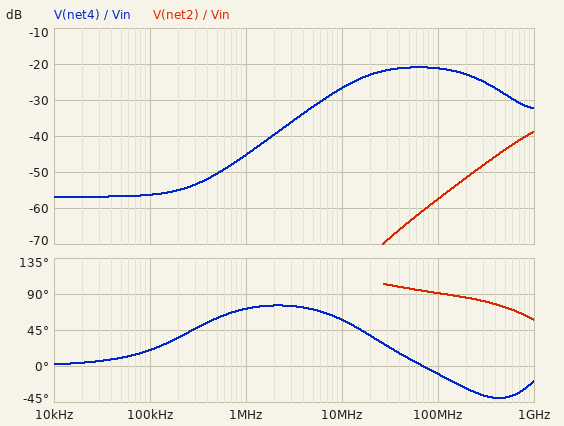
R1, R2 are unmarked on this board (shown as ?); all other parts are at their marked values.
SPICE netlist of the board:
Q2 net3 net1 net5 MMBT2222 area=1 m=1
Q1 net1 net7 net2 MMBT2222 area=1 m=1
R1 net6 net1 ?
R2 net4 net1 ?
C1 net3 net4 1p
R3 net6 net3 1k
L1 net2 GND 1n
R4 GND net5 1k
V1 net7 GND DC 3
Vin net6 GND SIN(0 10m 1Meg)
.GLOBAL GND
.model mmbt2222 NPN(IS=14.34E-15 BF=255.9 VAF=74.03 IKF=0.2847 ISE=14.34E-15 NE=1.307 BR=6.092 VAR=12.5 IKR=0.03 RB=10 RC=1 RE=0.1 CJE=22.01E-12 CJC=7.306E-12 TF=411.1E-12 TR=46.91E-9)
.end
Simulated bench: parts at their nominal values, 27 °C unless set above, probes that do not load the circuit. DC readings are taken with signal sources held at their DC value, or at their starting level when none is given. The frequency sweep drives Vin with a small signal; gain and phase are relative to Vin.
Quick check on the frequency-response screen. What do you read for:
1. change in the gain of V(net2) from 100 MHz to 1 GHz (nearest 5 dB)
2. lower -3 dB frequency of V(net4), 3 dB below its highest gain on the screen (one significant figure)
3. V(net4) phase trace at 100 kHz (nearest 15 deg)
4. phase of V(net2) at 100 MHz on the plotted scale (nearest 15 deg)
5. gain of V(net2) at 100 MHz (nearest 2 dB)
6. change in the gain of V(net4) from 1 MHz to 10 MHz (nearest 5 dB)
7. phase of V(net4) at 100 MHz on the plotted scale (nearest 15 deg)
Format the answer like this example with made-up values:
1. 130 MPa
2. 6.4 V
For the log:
1. 20 dB
2. 20 MHz
3. 15 deg
4. 90 deg
5. -58 dB
6. 20 dB
7. -15 deg
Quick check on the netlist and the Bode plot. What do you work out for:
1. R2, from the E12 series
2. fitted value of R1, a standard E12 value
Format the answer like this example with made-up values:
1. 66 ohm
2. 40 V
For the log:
1. 820 Ω
2. 820 Ω
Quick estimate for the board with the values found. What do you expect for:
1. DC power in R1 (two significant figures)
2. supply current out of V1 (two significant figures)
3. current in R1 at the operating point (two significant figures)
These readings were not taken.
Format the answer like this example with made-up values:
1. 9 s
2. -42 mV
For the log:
1. 2.3 µW
2. 210 mA
3. 53 µA
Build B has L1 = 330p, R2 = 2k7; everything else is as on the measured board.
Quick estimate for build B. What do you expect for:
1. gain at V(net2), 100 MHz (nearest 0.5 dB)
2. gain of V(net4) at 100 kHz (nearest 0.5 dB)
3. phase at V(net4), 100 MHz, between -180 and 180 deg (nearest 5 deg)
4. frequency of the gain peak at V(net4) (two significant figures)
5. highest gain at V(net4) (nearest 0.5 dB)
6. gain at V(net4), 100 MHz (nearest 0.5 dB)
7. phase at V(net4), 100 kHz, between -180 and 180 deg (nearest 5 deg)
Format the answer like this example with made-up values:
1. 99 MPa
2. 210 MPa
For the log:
1. -67.0 dB
2. -53.0 dB
3. -40 deg
4. 35 MHz
5. -12.5 dB
6. -15.5 dB
7. 50 deg
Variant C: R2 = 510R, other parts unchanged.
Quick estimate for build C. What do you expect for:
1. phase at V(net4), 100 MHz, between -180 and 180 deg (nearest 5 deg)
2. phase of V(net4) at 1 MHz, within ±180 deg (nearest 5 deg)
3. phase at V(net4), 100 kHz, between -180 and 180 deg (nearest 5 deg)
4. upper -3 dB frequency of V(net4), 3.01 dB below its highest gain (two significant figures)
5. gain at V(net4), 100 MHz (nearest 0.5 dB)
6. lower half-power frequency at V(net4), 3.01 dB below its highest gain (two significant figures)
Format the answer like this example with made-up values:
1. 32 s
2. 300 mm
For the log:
1. 0 deg
2. 65 deg
3. 15 deg
4. 380 MHz
5. -24.5 dB
6. 17 MHz
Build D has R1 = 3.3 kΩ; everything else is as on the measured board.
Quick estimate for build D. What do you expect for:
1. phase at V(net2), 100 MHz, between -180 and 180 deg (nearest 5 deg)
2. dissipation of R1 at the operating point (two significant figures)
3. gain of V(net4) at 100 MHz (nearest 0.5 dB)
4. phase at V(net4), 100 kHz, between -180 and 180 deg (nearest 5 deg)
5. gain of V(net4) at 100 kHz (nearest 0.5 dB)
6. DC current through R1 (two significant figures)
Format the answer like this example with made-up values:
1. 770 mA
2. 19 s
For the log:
1. 95 deg
2. 570 nW
3. -21.5 dB
4. 55 deg
5. -64.0 dB
6. 13 µA
